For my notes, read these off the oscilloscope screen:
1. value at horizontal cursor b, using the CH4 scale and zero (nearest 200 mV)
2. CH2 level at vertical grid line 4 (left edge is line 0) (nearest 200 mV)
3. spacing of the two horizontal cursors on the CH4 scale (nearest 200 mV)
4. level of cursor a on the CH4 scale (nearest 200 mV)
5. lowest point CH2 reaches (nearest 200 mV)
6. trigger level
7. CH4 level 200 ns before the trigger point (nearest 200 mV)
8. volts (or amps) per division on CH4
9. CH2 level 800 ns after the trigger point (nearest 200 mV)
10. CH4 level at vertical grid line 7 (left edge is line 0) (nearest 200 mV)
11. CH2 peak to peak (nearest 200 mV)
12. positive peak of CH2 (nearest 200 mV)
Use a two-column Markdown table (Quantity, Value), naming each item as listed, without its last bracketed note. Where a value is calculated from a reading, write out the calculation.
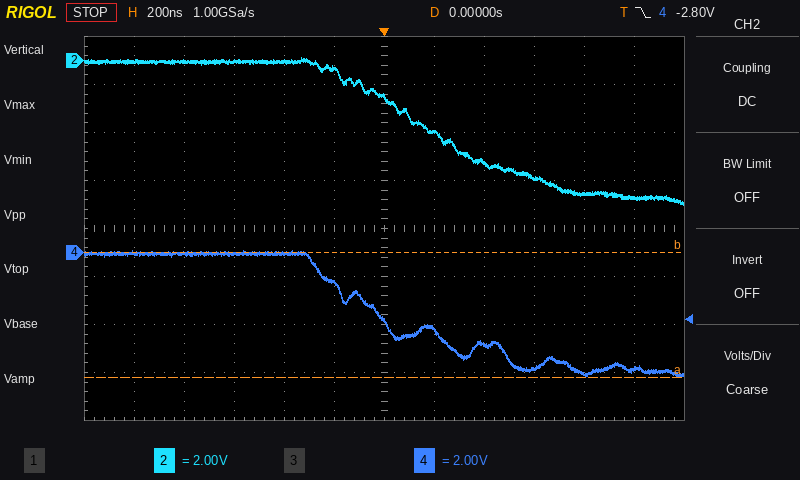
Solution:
| Quantity | Value |
|---|---|
| value at horizontal cursor b, using the CH4 scale and zero | 0.0 V |
| CH2 level at vertical grid line 4 (left edge is line 0) | 0.0 V |
| spacing of the two horizontal cursors on the CH4 scale | 5.2 V |
| level of cursor a on the CH4 scale | -5.2 V |
| lowest point CH2 reaches | -6.0 V |
| trigger level | -2.80 V |
| CH4 level 200 ns before the trigger point | -1.2 V |
| volts (or amps) per division on CH4 | 2 V |
| CH2 level 800 ns after the trigger point | -5.6 V |
| CH4 level at vertical grid line 7 (left edge is line 0) | -3.2 V |
| CH2 peak to peak | 200 mV − (-6.0 V) = 6.2 V |
| positive peak of CH2 | 200 mV |
